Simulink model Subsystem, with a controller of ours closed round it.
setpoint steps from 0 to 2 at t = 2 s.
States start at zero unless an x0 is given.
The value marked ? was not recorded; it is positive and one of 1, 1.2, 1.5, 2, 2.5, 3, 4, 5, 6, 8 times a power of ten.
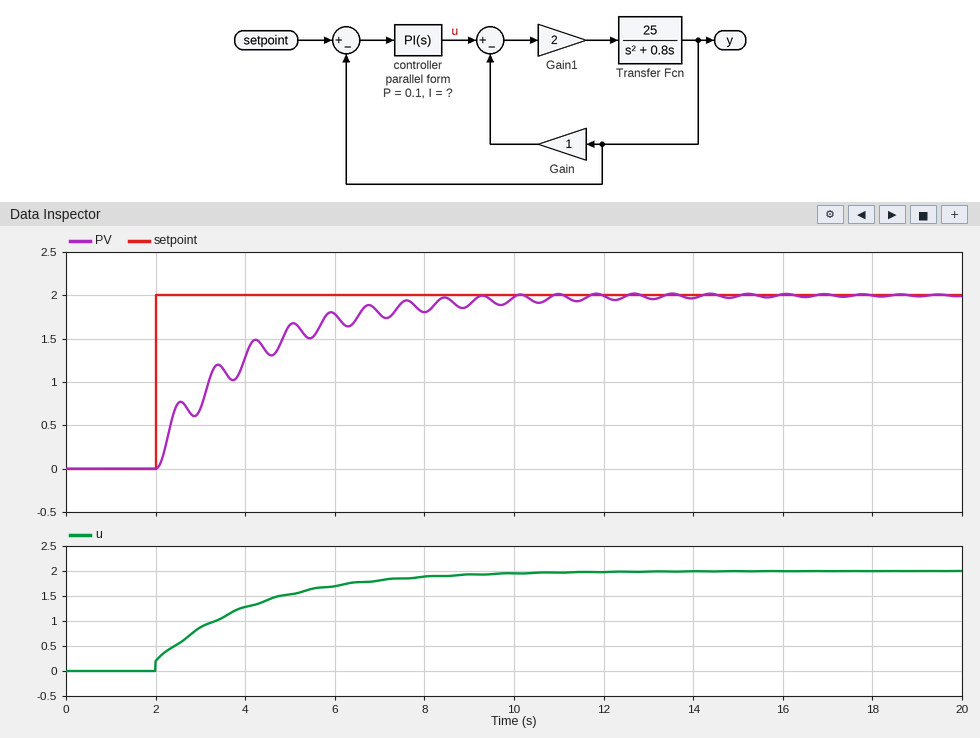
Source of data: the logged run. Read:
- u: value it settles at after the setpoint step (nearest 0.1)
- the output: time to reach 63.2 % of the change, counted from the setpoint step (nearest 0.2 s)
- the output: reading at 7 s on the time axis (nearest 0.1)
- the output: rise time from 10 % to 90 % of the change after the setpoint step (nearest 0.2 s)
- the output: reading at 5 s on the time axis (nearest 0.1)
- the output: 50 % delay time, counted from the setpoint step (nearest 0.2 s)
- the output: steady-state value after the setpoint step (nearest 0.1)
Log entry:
2.0
2.0 s
1.8
3.6 s
1.7
1.2 s
2.0
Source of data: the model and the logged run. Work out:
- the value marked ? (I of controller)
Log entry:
0.5
